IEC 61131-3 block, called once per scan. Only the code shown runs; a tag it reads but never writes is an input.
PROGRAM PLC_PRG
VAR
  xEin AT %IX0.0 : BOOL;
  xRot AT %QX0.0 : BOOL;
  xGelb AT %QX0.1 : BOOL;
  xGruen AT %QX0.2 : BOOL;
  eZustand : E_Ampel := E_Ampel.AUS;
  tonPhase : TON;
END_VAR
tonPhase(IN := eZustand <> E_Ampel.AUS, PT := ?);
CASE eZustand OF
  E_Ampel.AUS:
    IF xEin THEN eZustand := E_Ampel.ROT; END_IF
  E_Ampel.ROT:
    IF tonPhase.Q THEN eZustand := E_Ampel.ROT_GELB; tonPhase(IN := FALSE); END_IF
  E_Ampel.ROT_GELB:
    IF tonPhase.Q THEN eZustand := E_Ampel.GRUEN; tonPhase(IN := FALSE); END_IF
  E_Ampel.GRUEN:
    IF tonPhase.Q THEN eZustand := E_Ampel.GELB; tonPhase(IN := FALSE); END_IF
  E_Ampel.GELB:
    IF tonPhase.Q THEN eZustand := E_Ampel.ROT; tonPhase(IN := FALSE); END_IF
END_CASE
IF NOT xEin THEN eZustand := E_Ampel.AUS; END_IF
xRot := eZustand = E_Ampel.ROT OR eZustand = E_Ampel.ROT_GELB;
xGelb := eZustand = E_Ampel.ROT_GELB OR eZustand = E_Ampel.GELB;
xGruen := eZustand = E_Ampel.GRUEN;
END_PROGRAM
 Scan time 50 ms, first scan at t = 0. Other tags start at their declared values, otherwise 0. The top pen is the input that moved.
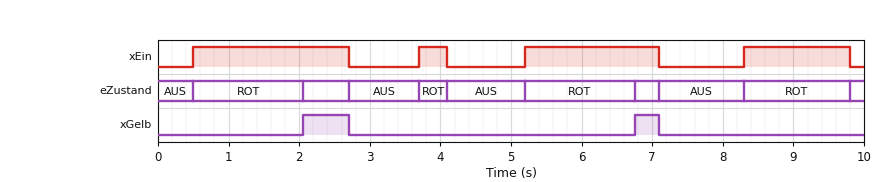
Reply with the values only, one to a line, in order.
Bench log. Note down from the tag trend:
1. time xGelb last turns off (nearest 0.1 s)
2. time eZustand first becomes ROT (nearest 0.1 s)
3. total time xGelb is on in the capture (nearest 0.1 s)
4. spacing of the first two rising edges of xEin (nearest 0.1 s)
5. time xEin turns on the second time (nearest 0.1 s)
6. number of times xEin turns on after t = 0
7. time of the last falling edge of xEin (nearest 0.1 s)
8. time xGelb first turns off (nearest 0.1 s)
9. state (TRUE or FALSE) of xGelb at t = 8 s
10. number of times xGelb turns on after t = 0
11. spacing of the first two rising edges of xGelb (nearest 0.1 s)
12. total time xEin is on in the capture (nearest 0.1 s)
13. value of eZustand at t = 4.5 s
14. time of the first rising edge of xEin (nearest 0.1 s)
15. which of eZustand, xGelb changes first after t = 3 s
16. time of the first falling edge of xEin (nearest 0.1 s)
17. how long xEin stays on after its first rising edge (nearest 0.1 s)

7.1 s
0.5 s
1.0 s
3.2 s
3.7 s
4
9.8 s
2.7 s
FALSE
2
4.7 s
6.0 s
AUS
0.5 s
eZustand
2.7 s
2.2 s
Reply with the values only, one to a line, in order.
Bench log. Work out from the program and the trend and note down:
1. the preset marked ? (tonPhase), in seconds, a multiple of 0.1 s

1.5 s
